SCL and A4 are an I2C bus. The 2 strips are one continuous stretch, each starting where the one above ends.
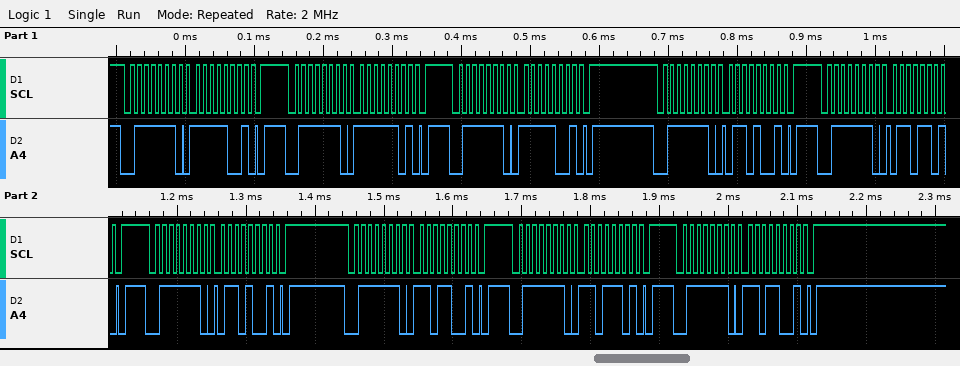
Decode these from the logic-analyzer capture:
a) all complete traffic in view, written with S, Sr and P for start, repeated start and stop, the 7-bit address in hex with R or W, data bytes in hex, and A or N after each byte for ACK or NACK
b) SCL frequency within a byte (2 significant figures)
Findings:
S 3FW A F9 A P S 3FW A FD A P S 3FW A F9 A P S 3FW A 69 A P S 3FW A 6D A P S 3FW A 69 A P S 3FW A D9 A P S 3FW A DD A P S 3FW A D9 A P
100 kHz
